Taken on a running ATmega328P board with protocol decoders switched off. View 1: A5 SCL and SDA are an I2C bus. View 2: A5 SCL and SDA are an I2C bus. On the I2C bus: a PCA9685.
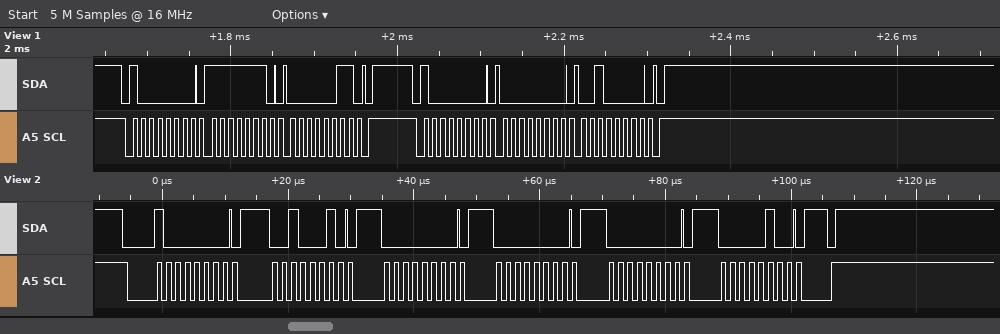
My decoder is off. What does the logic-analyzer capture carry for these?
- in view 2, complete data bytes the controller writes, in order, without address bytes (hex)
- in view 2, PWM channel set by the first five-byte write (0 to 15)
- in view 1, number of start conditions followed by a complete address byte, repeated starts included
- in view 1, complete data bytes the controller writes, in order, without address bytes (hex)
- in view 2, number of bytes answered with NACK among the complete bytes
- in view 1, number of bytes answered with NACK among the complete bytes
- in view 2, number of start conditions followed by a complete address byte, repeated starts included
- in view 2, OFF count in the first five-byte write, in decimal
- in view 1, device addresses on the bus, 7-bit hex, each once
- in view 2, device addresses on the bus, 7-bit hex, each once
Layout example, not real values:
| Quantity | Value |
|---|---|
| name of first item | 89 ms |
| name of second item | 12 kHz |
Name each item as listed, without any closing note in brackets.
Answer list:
| Quantity | Value |
|---|---|
| in view 2, complete data bytes the controller writes, in order, without address bytes | 22 00 00 00 04 |
| in view 2, PWM channel set by the first five-byte write | 7 |
| in view 1, number of start conditions followed by a complete address byte, repeated starts included | 2 |
| in view 1, complete data bytes the controller writes, in order, without address bytes | FE 03 00 20 |
| in view 2, number of bytes answered with NACK among the complete bytes | 0 |
| in view 1, number of bytes answered with NACK among the complete bytes | 0 |
| in view 2, number of start conditions followed by a complete address byte, repeated starts included | 1 |
| in view 2, OFF count in the first five-byte write, in decimal | 1024 |
| in view 1, device addresses on the bus, 7-bit hex, each once | 0x40 |
| in view 2, device addresses on the bus, 7-bit hex, each once | 0x40 |
